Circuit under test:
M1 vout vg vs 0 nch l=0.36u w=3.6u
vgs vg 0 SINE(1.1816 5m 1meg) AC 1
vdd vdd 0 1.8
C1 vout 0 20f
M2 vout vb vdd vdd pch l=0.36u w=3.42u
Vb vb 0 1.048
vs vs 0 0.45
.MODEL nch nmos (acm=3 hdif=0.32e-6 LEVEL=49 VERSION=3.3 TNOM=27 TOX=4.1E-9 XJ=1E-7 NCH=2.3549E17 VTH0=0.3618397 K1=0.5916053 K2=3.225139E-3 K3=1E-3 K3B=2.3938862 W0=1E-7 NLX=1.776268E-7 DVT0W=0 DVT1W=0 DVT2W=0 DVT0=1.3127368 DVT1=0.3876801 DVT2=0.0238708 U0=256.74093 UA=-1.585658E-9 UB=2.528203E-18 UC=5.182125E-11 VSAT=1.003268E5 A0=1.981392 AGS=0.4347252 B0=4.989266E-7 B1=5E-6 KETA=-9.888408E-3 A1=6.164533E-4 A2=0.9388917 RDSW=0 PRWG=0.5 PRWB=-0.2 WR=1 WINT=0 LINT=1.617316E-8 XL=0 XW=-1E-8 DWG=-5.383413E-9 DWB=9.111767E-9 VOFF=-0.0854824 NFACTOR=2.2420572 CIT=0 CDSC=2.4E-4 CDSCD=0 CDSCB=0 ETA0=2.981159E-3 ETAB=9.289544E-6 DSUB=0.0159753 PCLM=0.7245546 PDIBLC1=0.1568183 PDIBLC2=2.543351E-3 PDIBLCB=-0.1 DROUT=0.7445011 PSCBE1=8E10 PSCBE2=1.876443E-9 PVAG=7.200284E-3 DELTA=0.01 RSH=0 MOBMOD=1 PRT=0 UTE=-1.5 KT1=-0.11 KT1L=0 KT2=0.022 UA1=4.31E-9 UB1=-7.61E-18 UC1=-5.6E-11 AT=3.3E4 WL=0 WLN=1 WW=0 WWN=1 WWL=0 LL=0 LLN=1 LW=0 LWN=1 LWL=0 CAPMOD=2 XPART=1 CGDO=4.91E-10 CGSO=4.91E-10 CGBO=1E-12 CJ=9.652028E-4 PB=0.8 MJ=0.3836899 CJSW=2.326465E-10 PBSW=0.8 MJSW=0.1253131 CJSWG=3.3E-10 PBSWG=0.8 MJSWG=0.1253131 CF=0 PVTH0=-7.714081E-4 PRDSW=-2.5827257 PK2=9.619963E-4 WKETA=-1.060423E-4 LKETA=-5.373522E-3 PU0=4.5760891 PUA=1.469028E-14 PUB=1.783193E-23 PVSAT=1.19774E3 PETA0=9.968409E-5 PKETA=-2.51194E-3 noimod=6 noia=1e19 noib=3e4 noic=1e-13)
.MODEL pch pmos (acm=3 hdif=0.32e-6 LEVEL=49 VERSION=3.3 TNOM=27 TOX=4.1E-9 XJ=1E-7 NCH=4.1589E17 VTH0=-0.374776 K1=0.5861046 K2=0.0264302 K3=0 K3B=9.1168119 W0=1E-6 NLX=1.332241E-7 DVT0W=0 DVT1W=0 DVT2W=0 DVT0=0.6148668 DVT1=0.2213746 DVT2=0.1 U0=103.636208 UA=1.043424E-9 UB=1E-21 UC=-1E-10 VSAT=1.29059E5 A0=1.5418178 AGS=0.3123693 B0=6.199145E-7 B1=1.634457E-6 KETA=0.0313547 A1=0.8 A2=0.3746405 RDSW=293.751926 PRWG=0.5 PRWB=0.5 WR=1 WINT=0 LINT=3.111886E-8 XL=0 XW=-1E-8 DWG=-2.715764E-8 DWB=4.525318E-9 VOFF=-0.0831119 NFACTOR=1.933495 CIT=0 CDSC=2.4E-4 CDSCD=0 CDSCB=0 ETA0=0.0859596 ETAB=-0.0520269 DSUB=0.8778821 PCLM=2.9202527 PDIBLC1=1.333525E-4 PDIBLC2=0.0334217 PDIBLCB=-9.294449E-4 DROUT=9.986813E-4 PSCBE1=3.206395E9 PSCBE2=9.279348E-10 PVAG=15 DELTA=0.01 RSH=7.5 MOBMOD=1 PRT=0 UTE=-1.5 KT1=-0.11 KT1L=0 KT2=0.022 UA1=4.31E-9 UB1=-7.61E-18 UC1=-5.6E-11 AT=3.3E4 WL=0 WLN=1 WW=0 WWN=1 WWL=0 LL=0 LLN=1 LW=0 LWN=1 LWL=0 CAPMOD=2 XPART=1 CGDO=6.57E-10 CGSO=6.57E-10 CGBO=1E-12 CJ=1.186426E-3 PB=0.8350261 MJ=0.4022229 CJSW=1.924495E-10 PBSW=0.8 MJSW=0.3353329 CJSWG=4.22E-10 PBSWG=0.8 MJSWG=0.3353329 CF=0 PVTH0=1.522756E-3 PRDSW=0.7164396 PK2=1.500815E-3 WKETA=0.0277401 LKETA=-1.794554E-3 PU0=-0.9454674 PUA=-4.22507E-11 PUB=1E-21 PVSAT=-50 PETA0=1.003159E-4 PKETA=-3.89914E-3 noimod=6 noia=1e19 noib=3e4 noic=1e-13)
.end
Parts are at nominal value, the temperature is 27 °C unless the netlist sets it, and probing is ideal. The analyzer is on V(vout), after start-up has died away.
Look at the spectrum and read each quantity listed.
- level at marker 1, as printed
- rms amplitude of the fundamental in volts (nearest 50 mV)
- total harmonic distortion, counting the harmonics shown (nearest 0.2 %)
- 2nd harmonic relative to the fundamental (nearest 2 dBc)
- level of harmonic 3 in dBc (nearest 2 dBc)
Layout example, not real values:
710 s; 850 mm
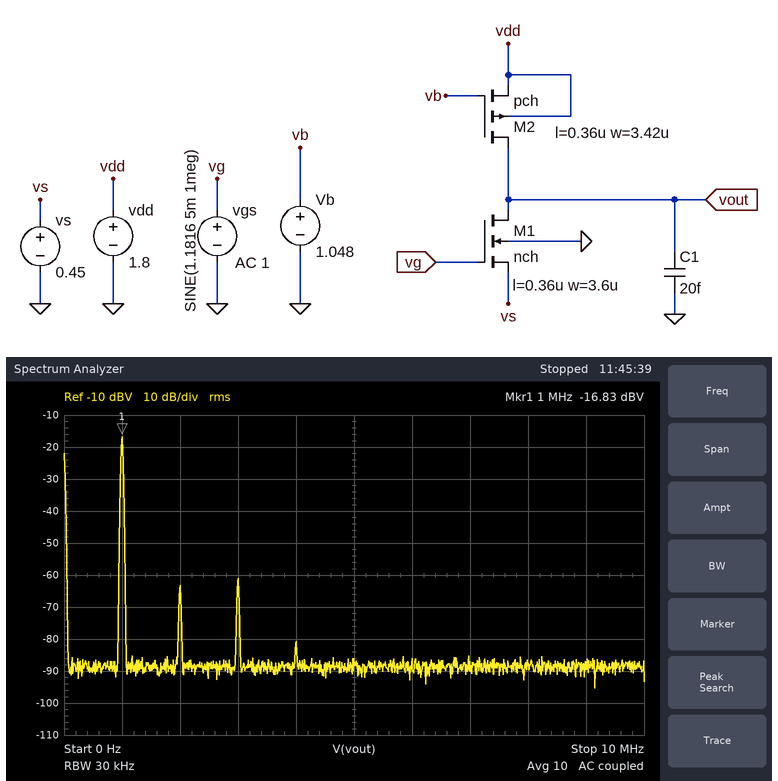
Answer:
-16.83 dBV; 150 mV; 0.8 %; -46 dBc; -44 dBc
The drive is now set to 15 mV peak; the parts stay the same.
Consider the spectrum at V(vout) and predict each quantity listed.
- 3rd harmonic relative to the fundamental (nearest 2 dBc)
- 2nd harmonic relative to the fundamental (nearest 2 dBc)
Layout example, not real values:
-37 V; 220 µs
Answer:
-22 dBc; -26 dBc
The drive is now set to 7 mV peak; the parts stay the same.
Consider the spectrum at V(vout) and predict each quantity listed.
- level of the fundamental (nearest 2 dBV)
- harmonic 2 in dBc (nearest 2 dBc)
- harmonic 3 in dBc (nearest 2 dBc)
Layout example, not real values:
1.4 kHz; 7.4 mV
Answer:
-14 dBV; -40 dBc; -38 dBc
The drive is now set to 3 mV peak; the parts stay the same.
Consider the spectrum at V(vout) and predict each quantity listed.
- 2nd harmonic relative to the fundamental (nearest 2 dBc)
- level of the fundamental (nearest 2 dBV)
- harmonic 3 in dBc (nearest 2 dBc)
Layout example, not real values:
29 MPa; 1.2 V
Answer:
-54 dBc; -22 dBV; -54 dBc
